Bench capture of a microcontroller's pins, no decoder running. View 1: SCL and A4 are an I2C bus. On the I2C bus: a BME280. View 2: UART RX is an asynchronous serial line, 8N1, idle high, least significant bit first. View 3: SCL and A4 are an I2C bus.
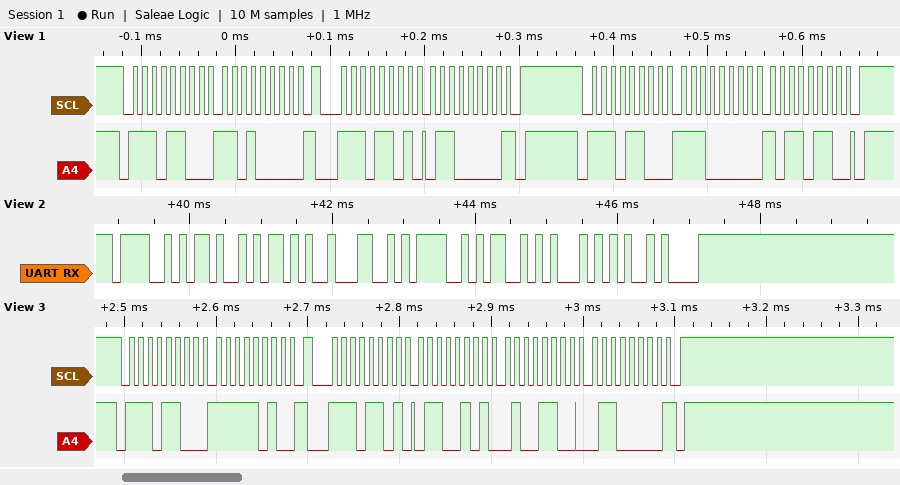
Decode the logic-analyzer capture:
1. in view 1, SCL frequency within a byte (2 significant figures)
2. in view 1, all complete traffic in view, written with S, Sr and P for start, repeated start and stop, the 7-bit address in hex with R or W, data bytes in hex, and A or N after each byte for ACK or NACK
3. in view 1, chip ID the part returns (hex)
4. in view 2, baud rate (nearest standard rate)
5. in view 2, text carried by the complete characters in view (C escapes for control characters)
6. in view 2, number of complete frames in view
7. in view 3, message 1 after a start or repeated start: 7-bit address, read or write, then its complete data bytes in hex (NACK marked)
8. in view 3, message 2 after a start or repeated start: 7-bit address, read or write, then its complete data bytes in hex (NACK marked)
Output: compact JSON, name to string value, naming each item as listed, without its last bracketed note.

{"in view 1, SCL frequency within a byte": "100 kHz", "in view 1, all complete traffic in view, written with S, Sr and P for start, repeated start and stop, the 7-bit address in hex with R or W, data bytes in hex, and A or N after each byte for ACK or NACK": "S 76W A D0 A Sr 76R A 60 N P S 76W A E0 A B6 A P", "in view 1, chip ID the part returns": "0x60", "in view 2, baud rate": "9600 baud", "in view 2, text carried by the complete characters in view": "\"OK+LOST\\n\"", "in view 2, number of complete frames in view": "8", "in view 3, message 1 after a start or repeated start: 7-bit address, read or write, then its complete data bytes in hex": "0x76 write: FA", "in view 3, message 2 after a start or repeated start: 7-bit address, read or write, then its complete data bytes in hex": "0x76 read: 65 4C 60 NACK"}
